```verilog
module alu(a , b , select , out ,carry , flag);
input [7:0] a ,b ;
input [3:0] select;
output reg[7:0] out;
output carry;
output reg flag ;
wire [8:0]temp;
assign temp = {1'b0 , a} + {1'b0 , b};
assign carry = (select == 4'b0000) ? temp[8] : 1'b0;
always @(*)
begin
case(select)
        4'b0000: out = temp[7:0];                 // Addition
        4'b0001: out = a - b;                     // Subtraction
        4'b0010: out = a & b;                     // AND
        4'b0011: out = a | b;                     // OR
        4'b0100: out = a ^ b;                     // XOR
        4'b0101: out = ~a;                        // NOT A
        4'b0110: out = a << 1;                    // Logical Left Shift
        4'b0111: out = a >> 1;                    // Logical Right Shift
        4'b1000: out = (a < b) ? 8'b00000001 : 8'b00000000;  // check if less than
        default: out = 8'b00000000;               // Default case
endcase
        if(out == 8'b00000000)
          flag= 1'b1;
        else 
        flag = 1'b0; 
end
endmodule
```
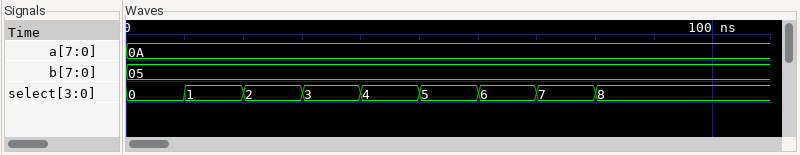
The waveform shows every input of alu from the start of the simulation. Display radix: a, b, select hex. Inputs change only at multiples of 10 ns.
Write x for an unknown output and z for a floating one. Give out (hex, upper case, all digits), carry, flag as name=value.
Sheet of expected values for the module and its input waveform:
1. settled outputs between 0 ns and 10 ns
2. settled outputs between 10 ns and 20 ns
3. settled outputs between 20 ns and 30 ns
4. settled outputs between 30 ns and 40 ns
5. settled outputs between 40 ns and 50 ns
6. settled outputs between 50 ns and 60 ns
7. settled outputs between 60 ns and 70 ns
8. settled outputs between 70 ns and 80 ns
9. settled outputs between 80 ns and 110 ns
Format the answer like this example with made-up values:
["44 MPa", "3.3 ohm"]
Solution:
["out=0F, carry=0, flag=0", "out=05, carry=0, flag=0", "out=00, carry=0, flag=1", "out=0F, carry=0, flag=0", "out=0F, carry=0, flag=0", "out=F5, carry=0, flag=0", "out=14, carry=0, flag=0", "out=05, carry=0, flag=0", "out=00, carry=0, flag=1"]
